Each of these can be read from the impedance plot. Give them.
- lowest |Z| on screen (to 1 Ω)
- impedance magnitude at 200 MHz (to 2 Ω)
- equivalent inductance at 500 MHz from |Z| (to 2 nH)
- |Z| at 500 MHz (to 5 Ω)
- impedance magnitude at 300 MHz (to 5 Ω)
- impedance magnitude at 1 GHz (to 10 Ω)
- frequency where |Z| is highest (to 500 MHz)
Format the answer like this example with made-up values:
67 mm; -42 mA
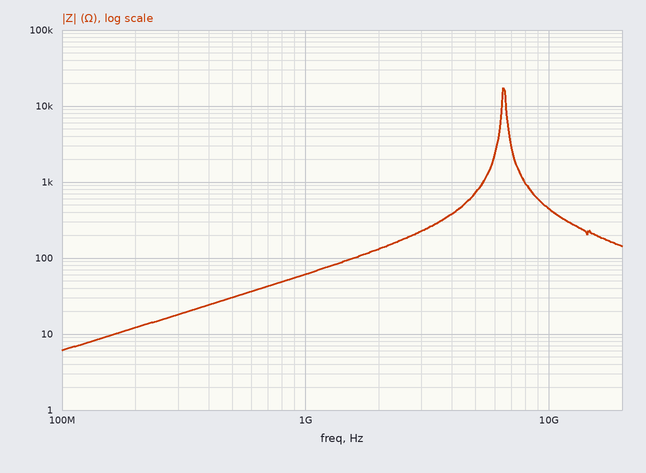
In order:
6 Ω; 12 Ω; 10 nH; 30 Ω; 20 Ω; 60 Ω; 6.5 GHz
